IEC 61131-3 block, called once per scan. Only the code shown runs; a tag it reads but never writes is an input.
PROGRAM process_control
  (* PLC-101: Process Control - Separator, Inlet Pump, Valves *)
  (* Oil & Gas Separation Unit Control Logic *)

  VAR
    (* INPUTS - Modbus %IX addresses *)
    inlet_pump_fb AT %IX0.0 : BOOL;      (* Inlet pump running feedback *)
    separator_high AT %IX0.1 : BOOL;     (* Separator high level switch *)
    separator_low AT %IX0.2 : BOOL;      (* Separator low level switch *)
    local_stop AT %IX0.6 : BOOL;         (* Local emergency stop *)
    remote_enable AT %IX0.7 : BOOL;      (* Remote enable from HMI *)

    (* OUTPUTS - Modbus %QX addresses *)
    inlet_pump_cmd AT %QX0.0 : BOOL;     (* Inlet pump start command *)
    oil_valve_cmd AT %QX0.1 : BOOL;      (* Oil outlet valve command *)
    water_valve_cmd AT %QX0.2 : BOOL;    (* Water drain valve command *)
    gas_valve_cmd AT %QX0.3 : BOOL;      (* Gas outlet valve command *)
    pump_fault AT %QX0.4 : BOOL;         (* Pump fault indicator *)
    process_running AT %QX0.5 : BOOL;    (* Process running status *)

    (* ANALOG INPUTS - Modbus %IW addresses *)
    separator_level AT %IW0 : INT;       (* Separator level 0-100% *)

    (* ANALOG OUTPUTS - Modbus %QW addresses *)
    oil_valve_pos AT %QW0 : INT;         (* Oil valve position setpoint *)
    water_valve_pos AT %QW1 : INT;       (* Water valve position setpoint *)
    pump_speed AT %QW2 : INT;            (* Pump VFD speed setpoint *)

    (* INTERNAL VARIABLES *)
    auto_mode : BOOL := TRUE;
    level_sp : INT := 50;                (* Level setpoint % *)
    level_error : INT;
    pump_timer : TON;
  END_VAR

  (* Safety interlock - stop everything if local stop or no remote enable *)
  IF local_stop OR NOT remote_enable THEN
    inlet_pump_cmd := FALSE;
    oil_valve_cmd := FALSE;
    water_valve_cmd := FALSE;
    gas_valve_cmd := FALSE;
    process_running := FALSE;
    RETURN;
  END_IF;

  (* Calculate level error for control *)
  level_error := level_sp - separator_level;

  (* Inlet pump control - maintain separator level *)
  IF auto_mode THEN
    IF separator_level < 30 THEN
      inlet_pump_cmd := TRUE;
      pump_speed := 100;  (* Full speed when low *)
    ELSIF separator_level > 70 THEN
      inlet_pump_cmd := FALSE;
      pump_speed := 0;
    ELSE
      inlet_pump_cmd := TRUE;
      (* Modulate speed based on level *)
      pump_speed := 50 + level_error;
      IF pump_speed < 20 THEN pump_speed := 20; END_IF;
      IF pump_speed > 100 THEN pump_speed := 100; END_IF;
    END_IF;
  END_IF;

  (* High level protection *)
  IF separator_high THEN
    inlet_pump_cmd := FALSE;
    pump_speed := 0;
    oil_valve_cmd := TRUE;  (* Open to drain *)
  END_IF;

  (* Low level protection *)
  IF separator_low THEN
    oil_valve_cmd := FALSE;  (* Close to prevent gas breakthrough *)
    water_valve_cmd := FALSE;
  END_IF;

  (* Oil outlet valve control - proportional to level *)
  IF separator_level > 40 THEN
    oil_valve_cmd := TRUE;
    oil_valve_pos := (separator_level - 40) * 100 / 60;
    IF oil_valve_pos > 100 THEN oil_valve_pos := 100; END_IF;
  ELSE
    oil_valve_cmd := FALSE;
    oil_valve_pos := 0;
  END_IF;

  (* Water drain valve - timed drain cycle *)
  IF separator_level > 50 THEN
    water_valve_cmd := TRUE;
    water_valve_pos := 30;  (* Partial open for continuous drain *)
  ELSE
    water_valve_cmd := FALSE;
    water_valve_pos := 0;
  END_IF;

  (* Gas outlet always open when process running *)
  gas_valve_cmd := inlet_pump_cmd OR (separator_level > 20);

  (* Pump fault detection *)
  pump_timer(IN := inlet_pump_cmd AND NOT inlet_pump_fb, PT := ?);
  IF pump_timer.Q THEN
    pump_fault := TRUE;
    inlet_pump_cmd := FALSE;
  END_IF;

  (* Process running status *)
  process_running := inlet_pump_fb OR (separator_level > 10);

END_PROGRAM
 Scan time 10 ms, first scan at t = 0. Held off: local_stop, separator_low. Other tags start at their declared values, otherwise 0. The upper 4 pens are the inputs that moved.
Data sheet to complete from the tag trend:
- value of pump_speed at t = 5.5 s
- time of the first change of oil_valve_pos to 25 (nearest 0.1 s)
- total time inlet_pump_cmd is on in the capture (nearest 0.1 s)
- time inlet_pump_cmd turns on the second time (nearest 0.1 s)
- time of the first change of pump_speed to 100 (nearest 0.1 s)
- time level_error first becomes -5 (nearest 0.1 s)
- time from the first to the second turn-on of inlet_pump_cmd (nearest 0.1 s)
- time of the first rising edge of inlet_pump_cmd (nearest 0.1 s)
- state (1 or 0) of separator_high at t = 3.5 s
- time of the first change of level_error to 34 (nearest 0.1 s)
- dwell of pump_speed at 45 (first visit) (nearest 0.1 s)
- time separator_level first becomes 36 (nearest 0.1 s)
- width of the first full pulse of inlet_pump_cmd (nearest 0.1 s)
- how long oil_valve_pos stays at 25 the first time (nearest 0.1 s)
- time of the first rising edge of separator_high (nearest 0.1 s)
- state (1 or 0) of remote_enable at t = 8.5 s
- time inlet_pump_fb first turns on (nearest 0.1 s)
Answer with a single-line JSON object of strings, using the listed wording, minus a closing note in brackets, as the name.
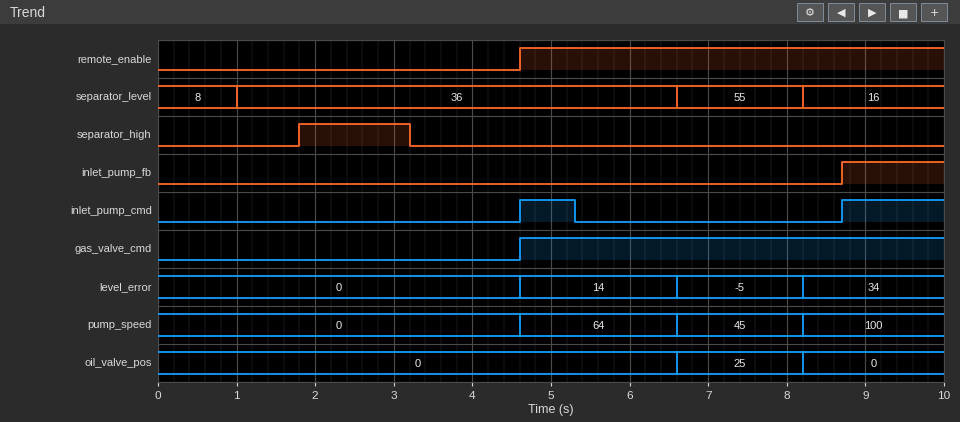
{"value of pump_speed at t = 5.5 s": "64", "time of the first change of oil_valve_pos to 25": "6.6 s", "total time inlet_pump_cmd is on in the capture": "2.0 s", "time inlet_pump_cmd turns on the second time": "8.7 s", "time of the first change of pump_speed to 100": "8.2 s", "time level_error first becomes -5": "6.6 s", "time from the first to the second turn-on of inlet_pump_cmd": "4.1 s", "time of the first rising edge of inlet_pump_cmd": "4.6 s", "state (1 or 0) of separator_high at t = 3.5 s": "0", "time of the first change of level_error to 34": "8.2 s", "dwell of pump_speed at 45 (first visit)": "1.6 s", "time separator_level first becomes 36": "1.0 s", "width of the first full pulse of inlet_pump_cmd": "0.7 s", "how long oil_valve_pos stays at 25 the first time": "1.6 s", "time of the first rising edge of separator_high": "1.8 s", "state (1 or 0) of remote_enable at t = 8.5 s": "1", "time inlet_pump_fb first turns on": "8.7 s"}
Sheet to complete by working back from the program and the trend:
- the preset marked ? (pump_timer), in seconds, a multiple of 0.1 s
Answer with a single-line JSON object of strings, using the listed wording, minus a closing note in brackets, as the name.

{"the preset marked ? (pump_timer), in seconds, a multiple of 0.1 s": "0.7 s"}
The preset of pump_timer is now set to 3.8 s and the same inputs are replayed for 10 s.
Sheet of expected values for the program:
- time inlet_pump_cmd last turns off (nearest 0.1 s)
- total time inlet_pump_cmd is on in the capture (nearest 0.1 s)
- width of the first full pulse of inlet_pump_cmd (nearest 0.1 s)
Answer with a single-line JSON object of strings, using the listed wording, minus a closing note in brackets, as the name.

{"time inlet_pump_cmd last turns off": "8.4 s", "total time inlet_pump_cmd is on in the capture": "5.1 s", "width of the first full pulse of inlet_pump_cmd": "3.8 s"}
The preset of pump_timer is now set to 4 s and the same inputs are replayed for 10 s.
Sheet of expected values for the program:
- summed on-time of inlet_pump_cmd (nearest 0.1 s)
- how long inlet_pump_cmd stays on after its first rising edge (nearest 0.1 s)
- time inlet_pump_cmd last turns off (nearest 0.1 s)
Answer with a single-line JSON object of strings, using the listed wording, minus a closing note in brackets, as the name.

{"summed on-time of inlet_pump_cmd": "5.3 s", "how long inlet_pump_cmd stays on after its first rising edge": "4.0 s", "time inlet_pump_cmd last turns off": "8.6 s"}
